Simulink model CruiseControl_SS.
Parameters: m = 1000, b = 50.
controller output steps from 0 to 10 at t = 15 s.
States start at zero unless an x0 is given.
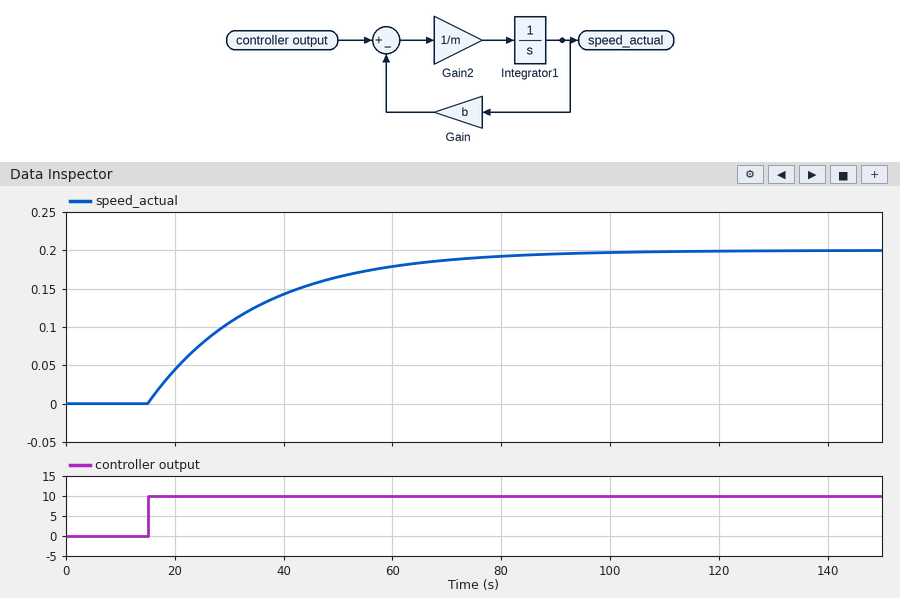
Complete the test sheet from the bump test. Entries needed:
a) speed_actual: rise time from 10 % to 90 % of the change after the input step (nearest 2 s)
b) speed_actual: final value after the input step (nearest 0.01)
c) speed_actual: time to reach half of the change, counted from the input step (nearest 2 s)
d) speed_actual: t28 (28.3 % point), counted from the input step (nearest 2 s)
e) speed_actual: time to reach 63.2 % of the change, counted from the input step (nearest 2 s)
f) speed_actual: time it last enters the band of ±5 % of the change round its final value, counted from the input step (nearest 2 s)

44 s
0.20
14 s
6 s
20 s
60 s
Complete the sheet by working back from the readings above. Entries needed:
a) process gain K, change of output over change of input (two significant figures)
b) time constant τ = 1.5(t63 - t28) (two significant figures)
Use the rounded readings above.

0.020
21 s
